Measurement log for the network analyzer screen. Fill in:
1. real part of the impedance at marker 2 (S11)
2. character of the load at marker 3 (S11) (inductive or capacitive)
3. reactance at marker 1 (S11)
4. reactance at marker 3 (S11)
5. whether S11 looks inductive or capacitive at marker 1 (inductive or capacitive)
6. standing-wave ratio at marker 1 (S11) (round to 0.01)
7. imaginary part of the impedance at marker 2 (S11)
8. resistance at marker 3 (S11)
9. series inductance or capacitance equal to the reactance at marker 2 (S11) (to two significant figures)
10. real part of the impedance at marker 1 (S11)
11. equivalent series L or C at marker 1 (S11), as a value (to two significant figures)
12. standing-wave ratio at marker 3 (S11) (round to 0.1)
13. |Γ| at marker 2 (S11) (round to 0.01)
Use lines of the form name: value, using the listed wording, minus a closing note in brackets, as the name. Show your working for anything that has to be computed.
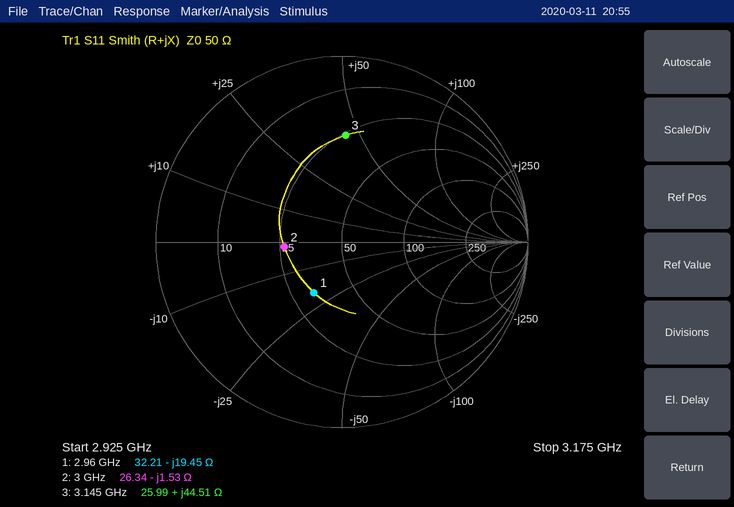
real part of the impedance at marker 2: 26.34 Ω
character of the load at marker 3 (S11): inductive
reactance at marker 1: -19.45 Ω
reactance at marker 3: +44.51 Ω
whether S11 looks inductive or capacitive at marker 1: capacitive
standing-wave ratio at marker 1 (S11): 1.91
imaginary part of the impedance at marker 2: -1.53 Ω
resistance at marker 3: 25.99 Ω
series inductance or capacitance equal to the reactance at marker 2 (S11): C = 1/(2π × 3 GHz × 1.53 Ω) ≈ 35 pF
real part of the impedance at marker 1: 32.21 Ω
equivalent series L or C at marker 1 (S11), as a value: C = 1/(2π × 2.96 GHz × 19.45 Ω) ≈ 2.8 pF
standing-wave ratio at marker 3 (S11): 3.7
|Γ| at marker 2 (S11): 0.31
